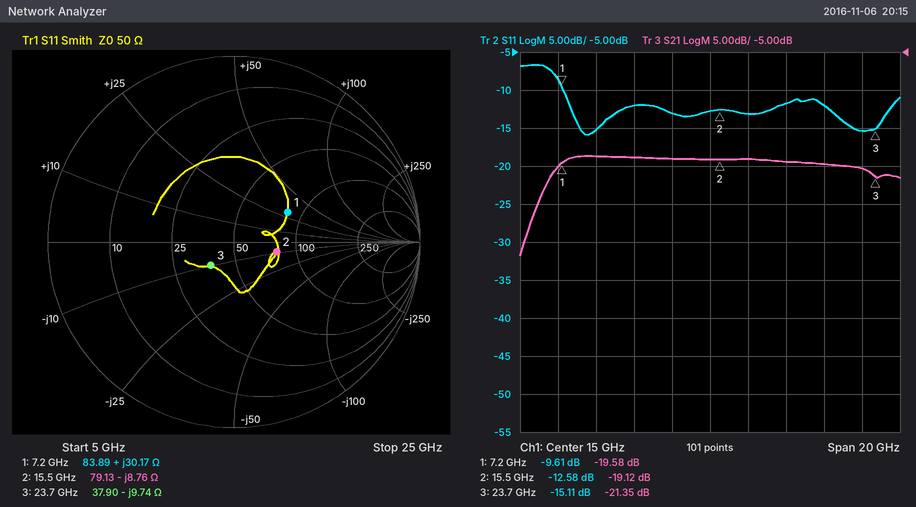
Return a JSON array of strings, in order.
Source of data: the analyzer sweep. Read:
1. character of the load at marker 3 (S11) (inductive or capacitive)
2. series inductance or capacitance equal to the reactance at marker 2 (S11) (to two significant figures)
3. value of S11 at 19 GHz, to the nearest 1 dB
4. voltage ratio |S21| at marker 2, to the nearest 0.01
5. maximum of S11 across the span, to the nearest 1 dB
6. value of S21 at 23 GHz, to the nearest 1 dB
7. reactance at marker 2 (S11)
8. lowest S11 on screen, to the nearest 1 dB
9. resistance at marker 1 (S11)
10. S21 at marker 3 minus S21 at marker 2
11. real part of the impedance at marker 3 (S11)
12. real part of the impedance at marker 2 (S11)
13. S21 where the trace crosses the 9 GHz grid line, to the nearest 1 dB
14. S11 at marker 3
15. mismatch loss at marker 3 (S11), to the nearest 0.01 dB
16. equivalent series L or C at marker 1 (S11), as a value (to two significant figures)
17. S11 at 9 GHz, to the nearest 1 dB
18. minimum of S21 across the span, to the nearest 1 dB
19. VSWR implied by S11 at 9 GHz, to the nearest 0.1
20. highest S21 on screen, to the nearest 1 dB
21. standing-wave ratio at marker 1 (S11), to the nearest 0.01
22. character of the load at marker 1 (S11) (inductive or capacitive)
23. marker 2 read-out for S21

["capacitive", "1.2 pF", "-12 dB", "0.11", "-7 dB", "-20 dB", "-8.76 Ω", "-16 dB", "83.89 Ω", "-2.23 dB", "37.90 Ω", "79.13 Ω", "-19 dB", "-15.11 dB", "0.14 dB", "670 pH", "-15 dB", "-32 dB", "1.4", "-19 dB", "1.99", "inductive", "-19.12 dB"]
